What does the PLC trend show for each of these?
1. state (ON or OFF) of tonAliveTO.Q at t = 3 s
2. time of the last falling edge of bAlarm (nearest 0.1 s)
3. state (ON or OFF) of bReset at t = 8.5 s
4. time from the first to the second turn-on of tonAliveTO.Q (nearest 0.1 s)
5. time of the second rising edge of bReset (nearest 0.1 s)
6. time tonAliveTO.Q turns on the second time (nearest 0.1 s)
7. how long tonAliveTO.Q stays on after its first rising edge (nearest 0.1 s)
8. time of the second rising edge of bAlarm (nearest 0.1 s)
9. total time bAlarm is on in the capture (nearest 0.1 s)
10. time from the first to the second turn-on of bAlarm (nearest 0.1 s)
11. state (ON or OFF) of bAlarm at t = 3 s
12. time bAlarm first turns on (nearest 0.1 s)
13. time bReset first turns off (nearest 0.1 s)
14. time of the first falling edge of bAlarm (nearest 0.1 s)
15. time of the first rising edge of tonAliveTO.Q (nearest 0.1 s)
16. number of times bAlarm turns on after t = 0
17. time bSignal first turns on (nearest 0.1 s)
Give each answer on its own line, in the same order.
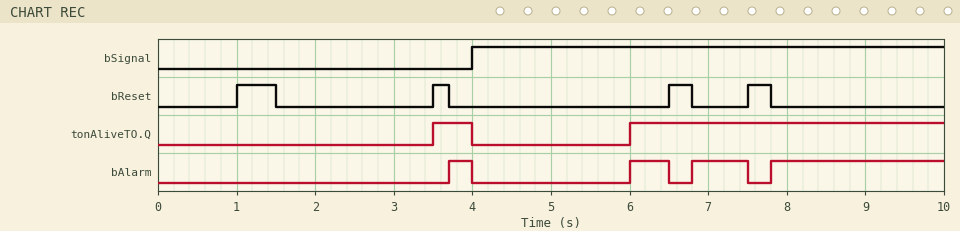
OFF
7.5 s
OFF
2.5 s
3.5 s
6.0 s
0.5 s
6.0 s
3.7 s
2.3 s
OFF
3.7 s
1.5 s
4.0 s
3.5 s
4
4.0 s
